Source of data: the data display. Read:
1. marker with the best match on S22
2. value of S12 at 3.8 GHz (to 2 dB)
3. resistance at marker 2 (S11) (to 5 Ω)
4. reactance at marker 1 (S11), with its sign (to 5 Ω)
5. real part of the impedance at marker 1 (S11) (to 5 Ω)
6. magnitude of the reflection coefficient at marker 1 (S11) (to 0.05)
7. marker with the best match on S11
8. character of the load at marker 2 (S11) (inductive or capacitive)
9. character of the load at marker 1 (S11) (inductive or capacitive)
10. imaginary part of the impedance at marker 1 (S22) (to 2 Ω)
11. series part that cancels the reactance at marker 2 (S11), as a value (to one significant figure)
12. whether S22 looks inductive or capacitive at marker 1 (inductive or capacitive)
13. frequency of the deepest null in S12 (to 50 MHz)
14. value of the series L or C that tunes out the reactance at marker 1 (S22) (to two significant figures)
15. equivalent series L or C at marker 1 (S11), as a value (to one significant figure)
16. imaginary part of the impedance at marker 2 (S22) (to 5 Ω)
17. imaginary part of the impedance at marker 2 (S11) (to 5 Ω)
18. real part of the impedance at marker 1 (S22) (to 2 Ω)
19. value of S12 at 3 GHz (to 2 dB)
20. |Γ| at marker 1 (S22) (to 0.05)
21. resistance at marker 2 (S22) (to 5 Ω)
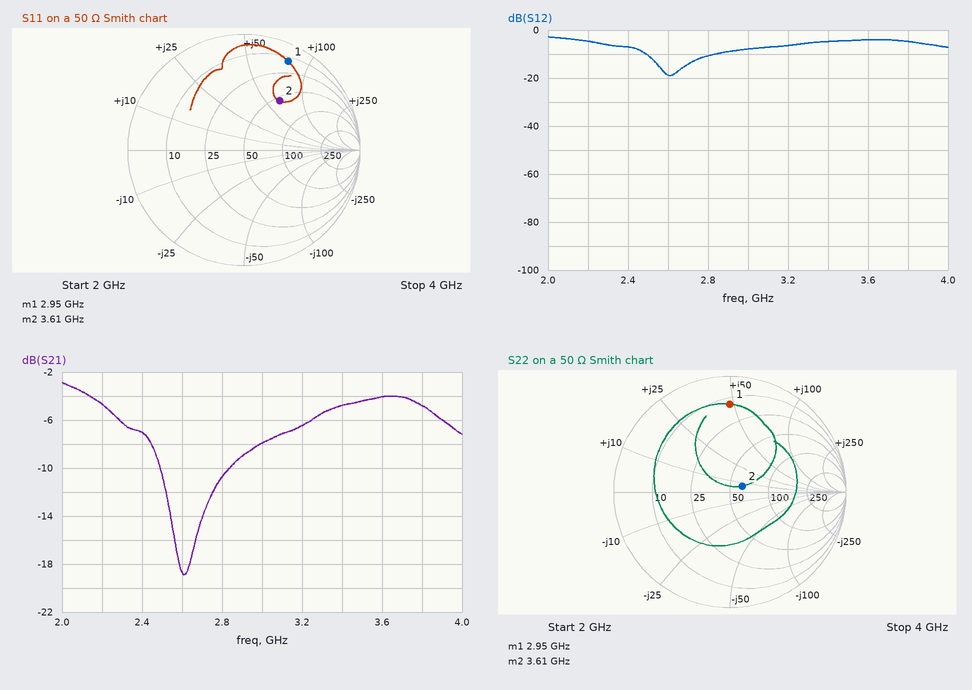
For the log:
marker 2
-4 dB
55 Ω
+80 Ω
15 Ω
0.85
marker 2
inductive
inductive
+48 Ω
700 fF
inductive
2.60 GHz
1.1 pF
4 nH
+5 Ω
+65 Ω
14 Ω
-8 dB
0.75
60 Ω
